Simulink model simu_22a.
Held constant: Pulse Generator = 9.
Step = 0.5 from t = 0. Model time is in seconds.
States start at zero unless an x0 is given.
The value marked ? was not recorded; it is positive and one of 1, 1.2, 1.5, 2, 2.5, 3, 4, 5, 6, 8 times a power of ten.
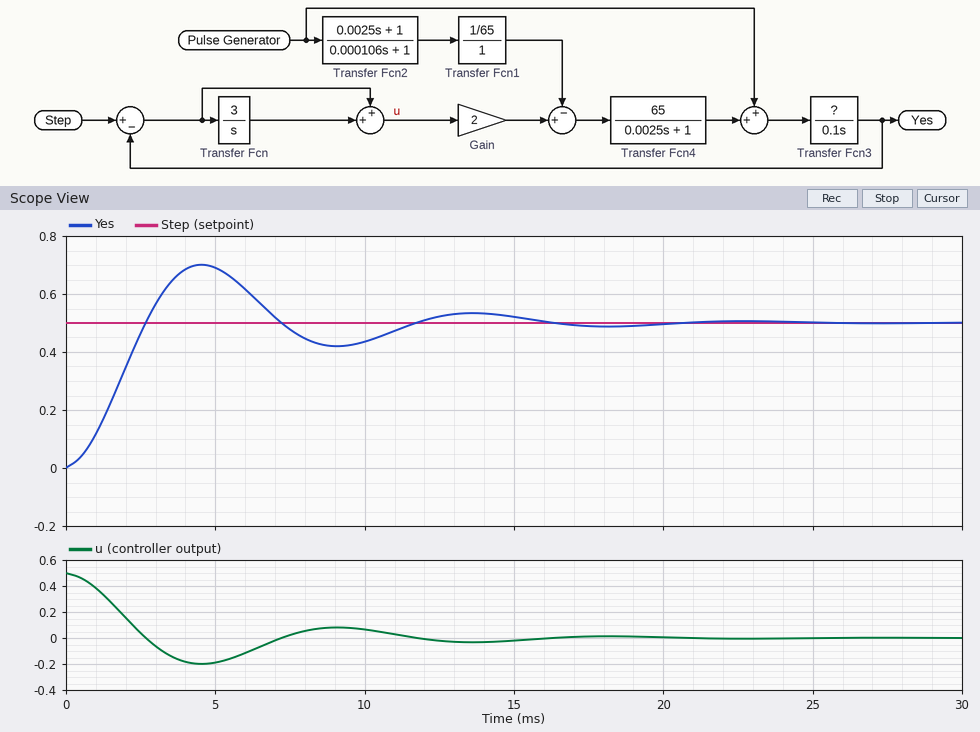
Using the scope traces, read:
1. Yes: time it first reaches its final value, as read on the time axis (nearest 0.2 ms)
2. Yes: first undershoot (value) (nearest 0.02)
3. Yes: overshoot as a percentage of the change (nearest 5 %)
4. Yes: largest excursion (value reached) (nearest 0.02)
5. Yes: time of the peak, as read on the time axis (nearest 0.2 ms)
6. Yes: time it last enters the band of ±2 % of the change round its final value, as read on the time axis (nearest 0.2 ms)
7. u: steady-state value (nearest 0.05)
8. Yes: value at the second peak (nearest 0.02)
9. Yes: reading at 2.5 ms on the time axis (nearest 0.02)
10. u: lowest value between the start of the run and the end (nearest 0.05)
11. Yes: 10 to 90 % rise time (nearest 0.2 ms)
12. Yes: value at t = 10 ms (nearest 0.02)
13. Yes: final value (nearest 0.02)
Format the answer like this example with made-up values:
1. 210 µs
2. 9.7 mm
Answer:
1. 2.6 ms
2. 0.42
3. 40 %
4. 0.70
5. 4.6 ms
6. 19.2 ms
7. 0.00
8. 0.54
9. 0.46
10. -0.20
11. 1.8 ms
12. 0.44
13. 0.50
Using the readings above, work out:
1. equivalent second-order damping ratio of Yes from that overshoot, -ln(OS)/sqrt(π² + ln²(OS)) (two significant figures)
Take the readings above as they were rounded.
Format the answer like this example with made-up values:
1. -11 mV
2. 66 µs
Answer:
1. 0.28
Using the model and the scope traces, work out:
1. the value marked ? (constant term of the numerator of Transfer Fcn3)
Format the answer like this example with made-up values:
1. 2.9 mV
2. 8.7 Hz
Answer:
1. 1
